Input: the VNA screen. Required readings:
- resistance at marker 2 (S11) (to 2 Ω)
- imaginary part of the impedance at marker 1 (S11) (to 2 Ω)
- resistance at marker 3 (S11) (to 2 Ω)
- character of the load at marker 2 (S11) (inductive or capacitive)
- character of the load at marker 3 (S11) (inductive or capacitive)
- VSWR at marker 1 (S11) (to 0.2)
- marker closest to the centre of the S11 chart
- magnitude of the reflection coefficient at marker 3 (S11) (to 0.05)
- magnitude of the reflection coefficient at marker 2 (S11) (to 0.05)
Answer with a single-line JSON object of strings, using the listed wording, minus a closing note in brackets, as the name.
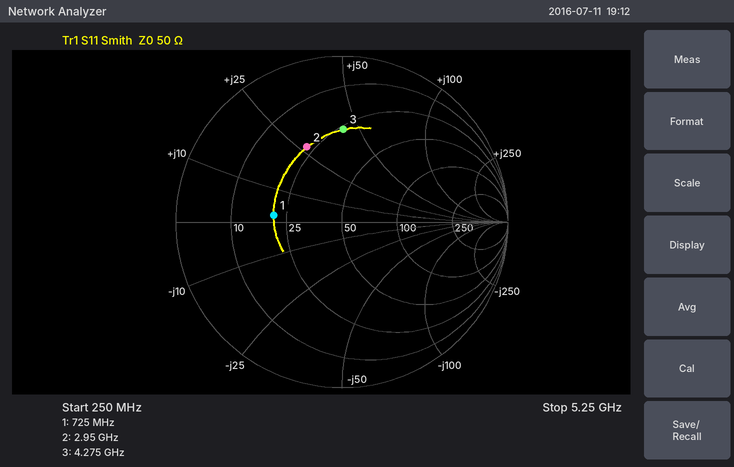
{"resistance at marker 2 (S11)": "22 Ω", "imaginary part of the impedance at marker 1 (S11)": "+2 Ω", "resistance at marker 3 (S11)": "26 Ω", "character of the load at marker 2 (S11)": "inductive", "character of the load at marker 3 (S11)": "inductive", "VSWR at marker 1 (S11)": "2.4", "marker closest to the centre of the S11 chart": "marker 1", "magnitude of the reflection coefficient at marker 3 (S11)": "0.55", "magnitude of the reflection coefficient at marker 2 (S11)": "0.50"}
